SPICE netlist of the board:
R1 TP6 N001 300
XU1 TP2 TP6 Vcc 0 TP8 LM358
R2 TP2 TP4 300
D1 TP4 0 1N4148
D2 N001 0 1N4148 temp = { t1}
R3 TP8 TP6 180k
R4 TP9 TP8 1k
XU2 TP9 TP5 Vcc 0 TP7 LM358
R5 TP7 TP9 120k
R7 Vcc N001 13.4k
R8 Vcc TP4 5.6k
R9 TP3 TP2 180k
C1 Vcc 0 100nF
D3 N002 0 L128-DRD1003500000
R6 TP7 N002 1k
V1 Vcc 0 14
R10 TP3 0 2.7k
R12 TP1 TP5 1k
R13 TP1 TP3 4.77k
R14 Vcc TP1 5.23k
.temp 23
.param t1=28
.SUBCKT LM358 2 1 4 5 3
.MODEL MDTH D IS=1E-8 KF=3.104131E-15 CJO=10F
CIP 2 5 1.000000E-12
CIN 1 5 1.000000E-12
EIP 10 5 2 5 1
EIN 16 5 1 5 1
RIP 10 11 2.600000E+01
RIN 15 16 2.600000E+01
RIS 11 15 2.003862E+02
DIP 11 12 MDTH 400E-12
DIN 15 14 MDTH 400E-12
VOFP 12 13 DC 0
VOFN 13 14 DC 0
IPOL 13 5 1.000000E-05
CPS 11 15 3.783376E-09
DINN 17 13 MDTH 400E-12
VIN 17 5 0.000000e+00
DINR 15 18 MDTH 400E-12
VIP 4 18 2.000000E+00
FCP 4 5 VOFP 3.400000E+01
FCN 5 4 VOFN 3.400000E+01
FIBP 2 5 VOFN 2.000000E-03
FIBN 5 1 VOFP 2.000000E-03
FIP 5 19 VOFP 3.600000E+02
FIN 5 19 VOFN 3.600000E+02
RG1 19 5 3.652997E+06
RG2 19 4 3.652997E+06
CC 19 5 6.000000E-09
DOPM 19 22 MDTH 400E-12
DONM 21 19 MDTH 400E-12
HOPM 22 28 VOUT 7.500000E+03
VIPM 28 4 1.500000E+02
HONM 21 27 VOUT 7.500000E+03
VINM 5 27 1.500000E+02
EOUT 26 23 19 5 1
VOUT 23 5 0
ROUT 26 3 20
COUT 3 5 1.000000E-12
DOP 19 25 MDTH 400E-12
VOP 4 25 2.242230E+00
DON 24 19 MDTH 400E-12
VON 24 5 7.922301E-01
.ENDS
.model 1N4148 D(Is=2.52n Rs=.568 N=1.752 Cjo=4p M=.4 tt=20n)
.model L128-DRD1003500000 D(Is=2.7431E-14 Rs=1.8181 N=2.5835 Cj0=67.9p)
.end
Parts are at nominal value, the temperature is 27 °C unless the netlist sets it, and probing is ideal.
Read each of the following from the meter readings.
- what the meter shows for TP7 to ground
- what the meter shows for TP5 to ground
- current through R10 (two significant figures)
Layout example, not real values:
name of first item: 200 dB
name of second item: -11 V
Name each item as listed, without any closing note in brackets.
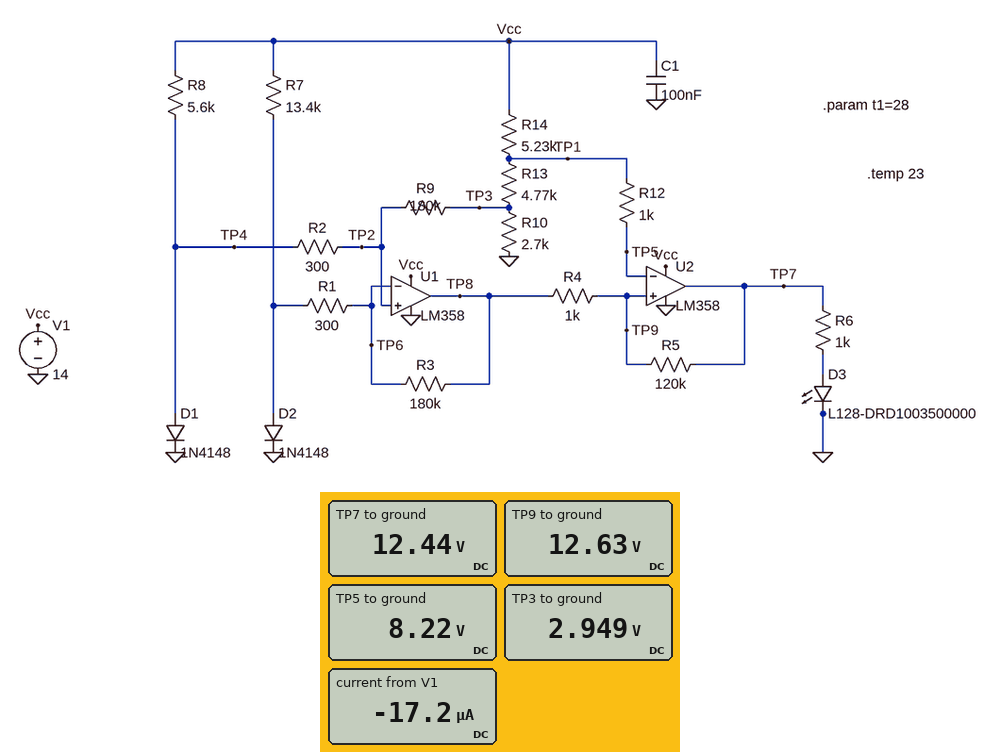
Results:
what the meter shows for TP7 to ground: 12.44 V
what the meter shows for TP5 to ground: 8.22 V
current through R10: 1.1 mA
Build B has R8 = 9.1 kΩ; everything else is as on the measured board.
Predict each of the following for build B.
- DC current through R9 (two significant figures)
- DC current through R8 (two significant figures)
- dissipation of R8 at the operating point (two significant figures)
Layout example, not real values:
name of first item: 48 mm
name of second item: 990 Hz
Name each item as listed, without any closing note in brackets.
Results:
DC current through R9: 13 µA
DC current through R8: 1.5 mA
dissipation of R8 at the operating point: 20 mW
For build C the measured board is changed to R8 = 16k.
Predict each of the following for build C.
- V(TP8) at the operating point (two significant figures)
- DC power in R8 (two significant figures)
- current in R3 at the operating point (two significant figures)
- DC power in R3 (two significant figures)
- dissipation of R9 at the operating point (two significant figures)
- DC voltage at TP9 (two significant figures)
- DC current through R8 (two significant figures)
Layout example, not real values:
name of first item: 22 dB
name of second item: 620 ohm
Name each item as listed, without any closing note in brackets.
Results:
V(TP8) at the operating point: 4.1 V
DC power in R8: 11 mW
current in R3 at the operating point: 19 µA
DC power in R3: 67 µW
dissipation of R9 at the operating point: 31 µW
DC voltage at TP9: 4.0 V
DC current through R8: 840 µA
